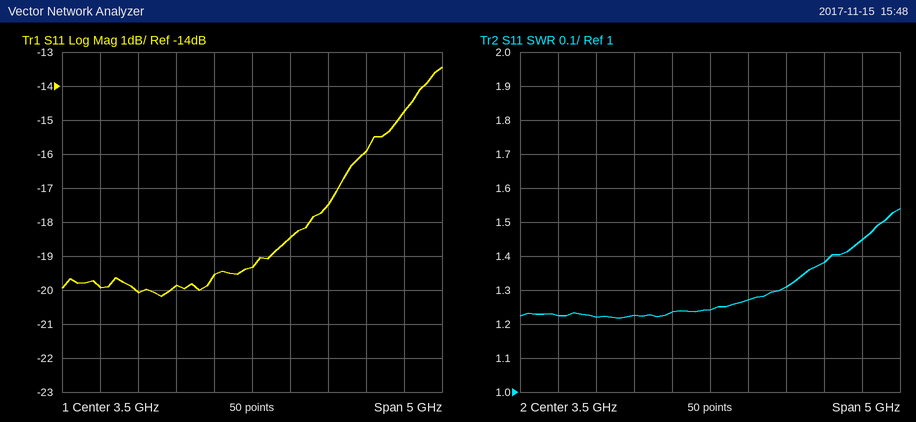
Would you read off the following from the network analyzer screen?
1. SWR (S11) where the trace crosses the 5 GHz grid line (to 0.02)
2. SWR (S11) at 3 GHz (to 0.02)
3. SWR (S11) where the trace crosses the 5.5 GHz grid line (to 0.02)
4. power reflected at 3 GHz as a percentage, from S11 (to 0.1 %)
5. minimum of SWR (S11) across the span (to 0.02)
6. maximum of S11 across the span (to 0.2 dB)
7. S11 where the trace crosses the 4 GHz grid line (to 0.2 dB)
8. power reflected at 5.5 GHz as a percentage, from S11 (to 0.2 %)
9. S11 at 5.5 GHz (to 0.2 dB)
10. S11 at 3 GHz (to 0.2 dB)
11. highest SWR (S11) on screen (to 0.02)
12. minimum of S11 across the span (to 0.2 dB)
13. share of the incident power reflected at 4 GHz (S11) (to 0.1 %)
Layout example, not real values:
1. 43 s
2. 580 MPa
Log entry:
1. 1.38
2. 1.24
3. 1.44
4. 1.1 %
5. 1.22
6. -13.4 dB
7. -18.4 dB
8. 3.4 %
9. -14.8 dB
10. -19.6 dB
11. 1.54
12. -20.2 dB
13. 1.4 %
